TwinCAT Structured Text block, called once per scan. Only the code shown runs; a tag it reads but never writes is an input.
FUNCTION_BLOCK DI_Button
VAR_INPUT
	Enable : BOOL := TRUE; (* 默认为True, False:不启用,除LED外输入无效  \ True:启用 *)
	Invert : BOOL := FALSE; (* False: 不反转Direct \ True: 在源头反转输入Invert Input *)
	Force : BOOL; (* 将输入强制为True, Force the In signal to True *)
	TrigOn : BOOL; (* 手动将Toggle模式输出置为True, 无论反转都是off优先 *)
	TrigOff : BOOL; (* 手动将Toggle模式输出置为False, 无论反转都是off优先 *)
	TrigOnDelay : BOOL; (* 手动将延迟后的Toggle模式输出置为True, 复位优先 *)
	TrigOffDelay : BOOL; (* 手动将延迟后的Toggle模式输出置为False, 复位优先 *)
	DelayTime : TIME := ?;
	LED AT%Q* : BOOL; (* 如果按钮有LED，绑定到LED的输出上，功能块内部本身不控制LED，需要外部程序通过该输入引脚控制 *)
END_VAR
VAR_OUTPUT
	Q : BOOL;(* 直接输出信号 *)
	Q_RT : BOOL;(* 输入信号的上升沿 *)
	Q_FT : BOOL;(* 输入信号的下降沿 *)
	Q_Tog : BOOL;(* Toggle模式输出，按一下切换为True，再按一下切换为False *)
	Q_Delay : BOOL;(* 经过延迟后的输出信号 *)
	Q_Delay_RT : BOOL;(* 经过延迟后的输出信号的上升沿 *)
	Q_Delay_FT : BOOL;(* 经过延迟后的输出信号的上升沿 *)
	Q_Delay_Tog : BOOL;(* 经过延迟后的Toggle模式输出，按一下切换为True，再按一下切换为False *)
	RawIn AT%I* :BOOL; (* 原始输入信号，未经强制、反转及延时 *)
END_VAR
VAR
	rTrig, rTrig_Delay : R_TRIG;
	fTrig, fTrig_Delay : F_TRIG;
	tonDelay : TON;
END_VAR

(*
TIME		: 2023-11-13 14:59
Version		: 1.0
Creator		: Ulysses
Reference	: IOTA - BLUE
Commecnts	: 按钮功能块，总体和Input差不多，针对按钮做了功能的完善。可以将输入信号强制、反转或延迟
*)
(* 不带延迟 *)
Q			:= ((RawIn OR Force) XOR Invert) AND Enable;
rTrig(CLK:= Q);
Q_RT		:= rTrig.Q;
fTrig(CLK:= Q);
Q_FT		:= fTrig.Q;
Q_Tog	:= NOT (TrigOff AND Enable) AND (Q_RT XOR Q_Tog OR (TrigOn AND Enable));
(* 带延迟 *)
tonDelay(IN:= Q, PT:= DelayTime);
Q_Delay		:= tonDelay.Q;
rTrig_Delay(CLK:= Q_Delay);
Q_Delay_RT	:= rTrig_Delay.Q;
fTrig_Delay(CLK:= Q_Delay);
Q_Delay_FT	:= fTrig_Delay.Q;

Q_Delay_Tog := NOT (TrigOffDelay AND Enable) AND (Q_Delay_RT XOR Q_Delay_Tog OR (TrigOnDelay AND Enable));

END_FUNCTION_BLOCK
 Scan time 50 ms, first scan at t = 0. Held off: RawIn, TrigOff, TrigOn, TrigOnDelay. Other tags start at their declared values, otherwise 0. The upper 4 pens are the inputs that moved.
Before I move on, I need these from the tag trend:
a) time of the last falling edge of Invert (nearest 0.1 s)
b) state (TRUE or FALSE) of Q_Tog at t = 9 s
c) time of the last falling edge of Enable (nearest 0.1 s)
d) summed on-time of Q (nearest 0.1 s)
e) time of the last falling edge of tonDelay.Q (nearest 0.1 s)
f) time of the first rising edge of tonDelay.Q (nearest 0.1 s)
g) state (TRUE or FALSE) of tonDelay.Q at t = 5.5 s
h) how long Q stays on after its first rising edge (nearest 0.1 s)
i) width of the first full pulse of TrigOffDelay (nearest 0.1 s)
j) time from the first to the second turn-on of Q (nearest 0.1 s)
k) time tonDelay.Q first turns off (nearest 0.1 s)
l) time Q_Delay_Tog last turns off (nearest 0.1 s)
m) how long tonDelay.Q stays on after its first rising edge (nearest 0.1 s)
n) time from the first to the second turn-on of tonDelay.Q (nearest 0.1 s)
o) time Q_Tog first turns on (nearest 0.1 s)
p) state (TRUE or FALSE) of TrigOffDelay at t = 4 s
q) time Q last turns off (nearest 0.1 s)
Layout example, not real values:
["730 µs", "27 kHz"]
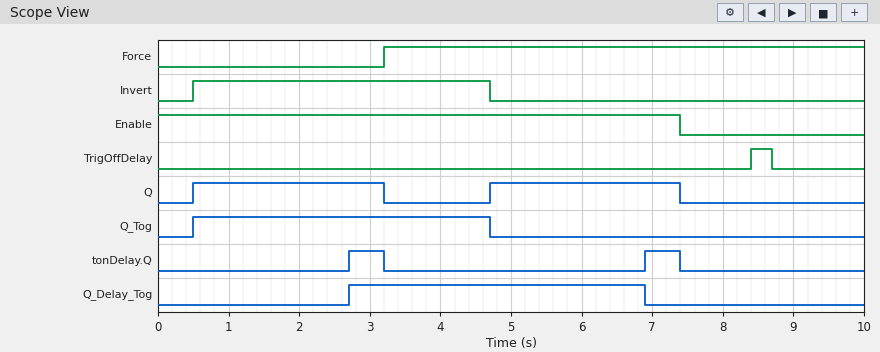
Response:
["4.7 s", "FALSE", "7.4 s", "5.4 s", "7.4 s", "2.7 s", "FALSE", "2.7 s", "0.3 s", "4.2 s", "3.2 s", "6.9 s", "0.5 s", "4.2 s", "0.5 s", "FALSE", "7.4 s"]
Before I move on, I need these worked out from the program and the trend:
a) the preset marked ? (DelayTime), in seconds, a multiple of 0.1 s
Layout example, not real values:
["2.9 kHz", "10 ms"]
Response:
["2.2 s"]
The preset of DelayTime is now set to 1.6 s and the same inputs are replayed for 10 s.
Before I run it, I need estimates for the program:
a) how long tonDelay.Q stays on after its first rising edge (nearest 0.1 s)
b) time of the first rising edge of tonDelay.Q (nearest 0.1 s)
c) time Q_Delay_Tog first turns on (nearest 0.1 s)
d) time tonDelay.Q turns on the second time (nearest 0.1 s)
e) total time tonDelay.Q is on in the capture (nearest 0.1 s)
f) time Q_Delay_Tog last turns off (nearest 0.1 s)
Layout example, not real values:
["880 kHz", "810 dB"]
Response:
["1.1 s", "2.1 s", "2.1 s", "6.3 s", "2.2 s", "6.3 s"]
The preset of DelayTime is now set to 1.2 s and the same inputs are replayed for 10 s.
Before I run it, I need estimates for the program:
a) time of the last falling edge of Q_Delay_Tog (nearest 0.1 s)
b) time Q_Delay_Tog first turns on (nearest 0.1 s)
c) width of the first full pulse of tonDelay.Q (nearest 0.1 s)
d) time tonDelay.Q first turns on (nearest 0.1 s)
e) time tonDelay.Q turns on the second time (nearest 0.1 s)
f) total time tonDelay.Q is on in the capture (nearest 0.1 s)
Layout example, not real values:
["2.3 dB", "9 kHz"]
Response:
["5.9 s", "1.7 s", "1.5 s", "1.7 s", "5.9 s", "3.0 s"]
